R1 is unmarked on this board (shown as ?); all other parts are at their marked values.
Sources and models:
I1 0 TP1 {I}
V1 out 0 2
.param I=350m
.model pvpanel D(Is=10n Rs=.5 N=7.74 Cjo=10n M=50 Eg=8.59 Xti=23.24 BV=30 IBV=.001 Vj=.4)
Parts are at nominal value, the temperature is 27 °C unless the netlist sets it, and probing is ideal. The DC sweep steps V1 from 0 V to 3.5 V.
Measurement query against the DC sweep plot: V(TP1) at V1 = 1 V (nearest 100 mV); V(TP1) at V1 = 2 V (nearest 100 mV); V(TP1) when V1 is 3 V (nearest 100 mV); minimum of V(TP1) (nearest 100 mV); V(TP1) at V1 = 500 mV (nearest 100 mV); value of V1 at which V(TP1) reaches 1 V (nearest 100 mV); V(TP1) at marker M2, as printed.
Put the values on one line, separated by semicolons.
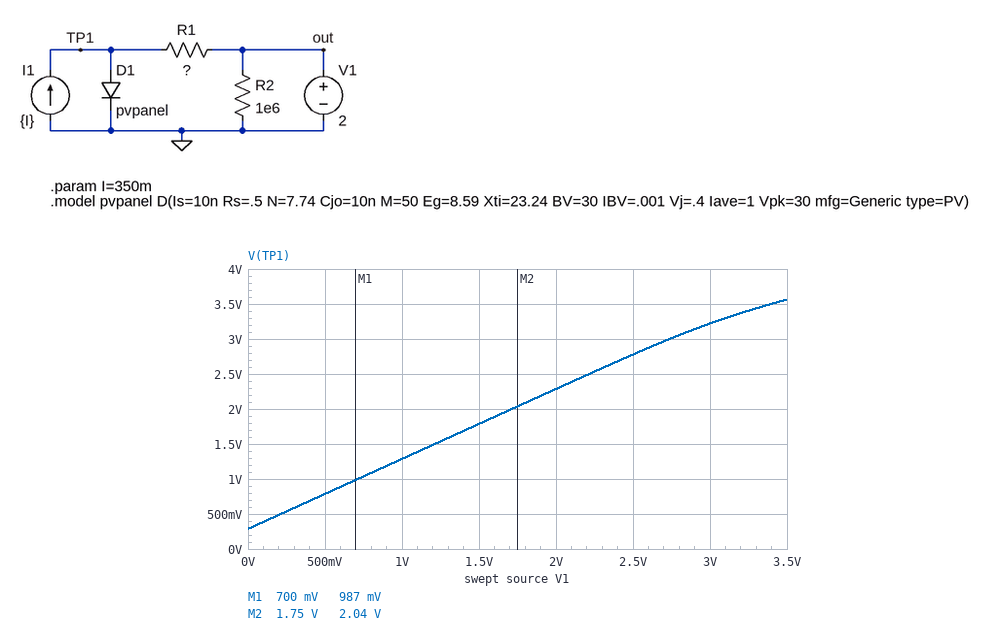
1.3 V; 2.3 V; 3.2 V; 300 mV; 800 mV; 700 mV; 2.04 V
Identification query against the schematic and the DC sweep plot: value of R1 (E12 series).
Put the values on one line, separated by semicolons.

0.82 Ω
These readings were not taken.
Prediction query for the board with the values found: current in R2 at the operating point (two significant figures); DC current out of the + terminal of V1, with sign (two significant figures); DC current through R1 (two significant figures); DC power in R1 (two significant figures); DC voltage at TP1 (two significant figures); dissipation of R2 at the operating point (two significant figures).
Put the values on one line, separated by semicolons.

2.0 µA; -350 mA; 350 mA; 100 mW; 2.3 V; 4.0 µW
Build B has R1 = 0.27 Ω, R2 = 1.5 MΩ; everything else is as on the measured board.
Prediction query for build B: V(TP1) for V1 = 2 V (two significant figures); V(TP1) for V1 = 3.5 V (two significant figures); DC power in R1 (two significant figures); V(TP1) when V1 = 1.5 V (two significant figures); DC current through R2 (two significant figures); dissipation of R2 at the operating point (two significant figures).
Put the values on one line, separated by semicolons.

2.1 V; 3.5 V; 33 mW; 1.6 V; 1.3 µA; 2.7 µW
